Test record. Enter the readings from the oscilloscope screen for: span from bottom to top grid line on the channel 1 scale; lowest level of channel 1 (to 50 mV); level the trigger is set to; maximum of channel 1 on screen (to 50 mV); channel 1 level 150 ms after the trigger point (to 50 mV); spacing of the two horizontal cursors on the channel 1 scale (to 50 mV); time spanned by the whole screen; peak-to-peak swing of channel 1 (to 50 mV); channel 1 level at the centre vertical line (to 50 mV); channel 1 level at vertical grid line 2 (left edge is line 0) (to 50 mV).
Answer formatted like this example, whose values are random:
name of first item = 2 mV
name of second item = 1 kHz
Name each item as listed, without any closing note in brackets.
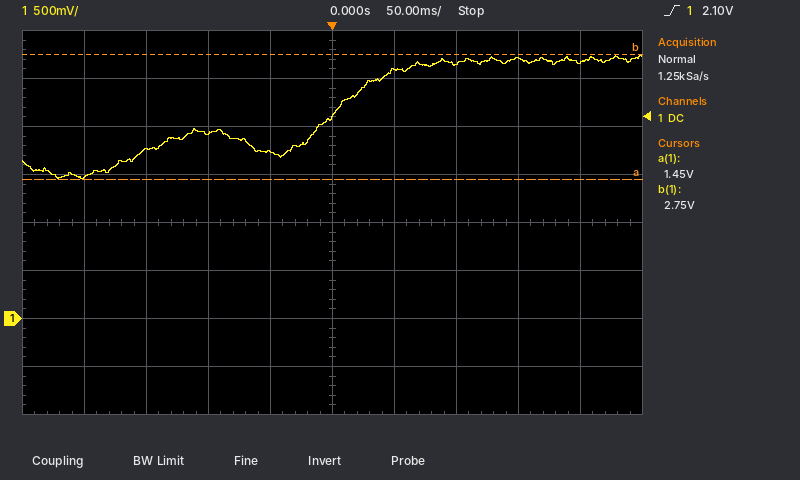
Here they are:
span from bottom to top grid line on the channel 1 scale = 4 V
lowest level of channel 1 = 1.45 V
level the trigger is set to = 2.10 V
maximum of channel 1 on screen = 2.75 V
channel 1 level 150 ms after the trigger point = 2.70 V
spacing of the two horizontal cursors on the channel 1 scale = 1.30 V
time spanned by the whole screen = 500 ms
peak-to-peak swing of channel 1 = 1.30 V
channel 1 level at the centre vertical line = 2.10 V
channel 1 level at vertical grid line 2 (left edge is line 0) = 1.75 V
